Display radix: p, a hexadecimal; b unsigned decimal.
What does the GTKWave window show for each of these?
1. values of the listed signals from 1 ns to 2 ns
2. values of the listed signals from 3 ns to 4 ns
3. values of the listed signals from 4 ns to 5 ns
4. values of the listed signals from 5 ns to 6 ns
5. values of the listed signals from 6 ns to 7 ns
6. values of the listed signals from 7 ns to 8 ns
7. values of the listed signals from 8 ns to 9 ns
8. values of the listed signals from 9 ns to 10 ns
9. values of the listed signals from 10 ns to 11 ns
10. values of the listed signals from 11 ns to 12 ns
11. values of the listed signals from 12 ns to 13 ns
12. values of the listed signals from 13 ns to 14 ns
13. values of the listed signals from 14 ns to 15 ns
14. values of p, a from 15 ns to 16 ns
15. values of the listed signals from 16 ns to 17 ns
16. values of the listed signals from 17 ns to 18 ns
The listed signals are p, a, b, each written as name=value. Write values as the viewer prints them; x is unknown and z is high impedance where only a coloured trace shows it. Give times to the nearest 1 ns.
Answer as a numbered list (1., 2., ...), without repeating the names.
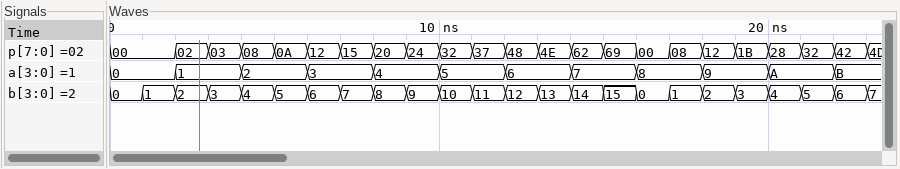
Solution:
1. p=00, a=0, b=1
2. p=03, a=1, b=3
3. p=08, a=2, b=4
4. p=0A, a=2, b=5
5. p=12, a=3, b=6
6. p=15, a=3, b=7
7. p=20, a=4, b=8
8. p=24, a=4, b=9
9. p=32, a=5, b=10
10. p=37, a=5, b=11
11. p=48, a=6, b=12
12. p=4E, a=6, b=13
13. p=62, a=7, b=14
14. p=69, a=7
15. p=00, a=8, b=0
16. p=08, a=8, b=1
